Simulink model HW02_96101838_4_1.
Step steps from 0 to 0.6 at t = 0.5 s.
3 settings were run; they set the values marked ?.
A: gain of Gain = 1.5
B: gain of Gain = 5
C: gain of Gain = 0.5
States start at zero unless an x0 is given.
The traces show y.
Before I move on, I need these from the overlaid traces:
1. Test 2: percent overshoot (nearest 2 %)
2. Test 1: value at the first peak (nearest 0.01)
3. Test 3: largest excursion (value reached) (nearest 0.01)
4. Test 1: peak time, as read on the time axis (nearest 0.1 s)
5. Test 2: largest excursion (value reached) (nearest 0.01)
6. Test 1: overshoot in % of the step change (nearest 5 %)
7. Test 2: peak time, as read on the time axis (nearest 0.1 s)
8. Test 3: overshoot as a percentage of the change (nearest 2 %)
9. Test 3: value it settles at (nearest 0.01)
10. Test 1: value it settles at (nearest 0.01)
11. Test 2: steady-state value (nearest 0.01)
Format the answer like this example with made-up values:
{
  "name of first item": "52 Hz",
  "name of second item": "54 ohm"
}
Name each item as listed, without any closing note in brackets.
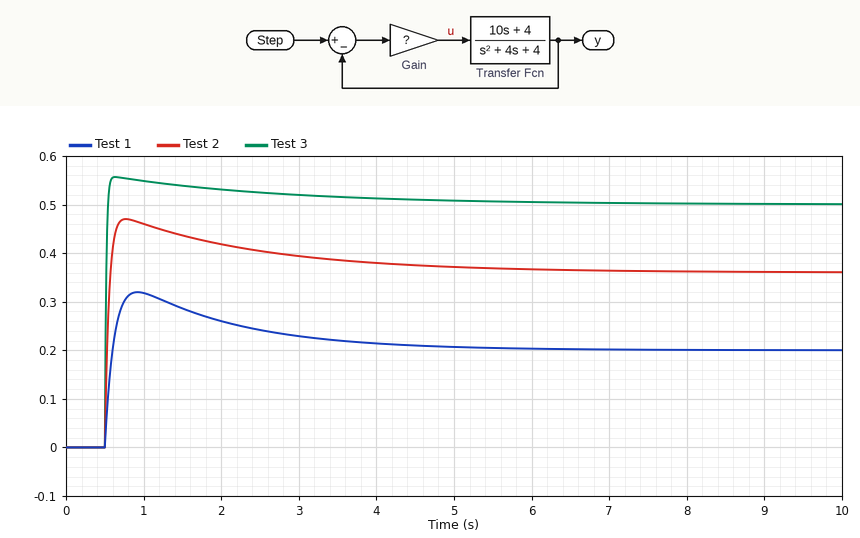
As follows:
{
  "Test 2: percent overshoot": "30 %",
  "Test 1: value at the first peak": "0.32",
  "Test 3: largest excursion (value reached)": "0.56",
  "Test 1: peak time, as read on the time axis": "0.9 s",
  "Test 2: largest excursion (value reached)": "0.47",
  "Test 1: overshoot in % of the step change": "60 %",
  "Test 2: peak time, as read on the time axis": "0.8 s",
  "Test 3: overshoot as a percentage of the change": "12 %",
  "Test 3: value it settles at": "0.50",
  "Test 1: value it settles at": "0.20",
  "Test 2: steady-state value": "0.36"
}
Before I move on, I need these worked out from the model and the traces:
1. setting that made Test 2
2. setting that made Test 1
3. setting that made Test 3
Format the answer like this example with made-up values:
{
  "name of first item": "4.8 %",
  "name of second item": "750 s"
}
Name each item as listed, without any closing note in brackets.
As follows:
{
  "setting that made Test 2": "A",
  "setting that made Test 1": "C",
  "setting that made Test 3": "B"
}
